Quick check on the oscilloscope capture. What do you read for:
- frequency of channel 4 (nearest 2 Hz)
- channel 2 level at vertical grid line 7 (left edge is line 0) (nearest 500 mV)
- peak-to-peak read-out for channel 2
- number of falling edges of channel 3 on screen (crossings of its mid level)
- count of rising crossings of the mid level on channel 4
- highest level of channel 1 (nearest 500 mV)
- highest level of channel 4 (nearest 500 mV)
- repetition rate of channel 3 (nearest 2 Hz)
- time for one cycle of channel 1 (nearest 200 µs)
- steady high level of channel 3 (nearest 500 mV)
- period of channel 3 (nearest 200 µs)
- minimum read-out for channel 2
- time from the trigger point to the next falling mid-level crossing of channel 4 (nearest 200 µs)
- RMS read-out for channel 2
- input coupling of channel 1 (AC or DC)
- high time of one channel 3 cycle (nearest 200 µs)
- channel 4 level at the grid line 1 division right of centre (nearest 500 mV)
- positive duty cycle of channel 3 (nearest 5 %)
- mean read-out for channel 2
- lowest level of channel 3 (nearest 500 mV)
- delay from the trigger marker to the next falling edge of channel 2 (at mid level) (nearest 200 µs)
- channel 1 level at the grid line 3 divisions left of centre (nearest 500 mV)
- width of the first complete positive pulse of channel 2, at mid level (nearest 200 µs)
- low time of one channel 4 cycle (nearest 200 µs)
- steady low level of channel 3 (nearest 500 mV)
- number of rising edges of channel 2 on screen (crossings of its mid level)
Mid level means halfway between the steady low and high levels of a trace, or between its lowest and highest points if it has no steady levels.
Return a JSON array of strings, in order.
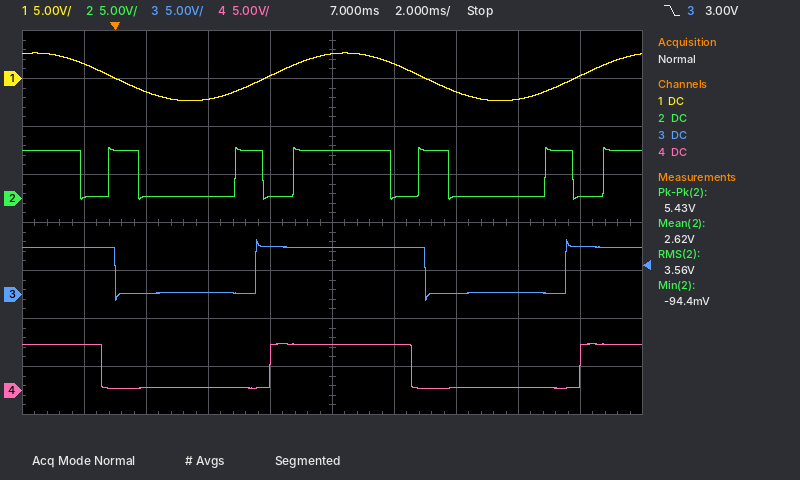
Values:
["100 Hz", "0.0 V", "5.43 V", "2", "2", "2.5 V", "5.0 V", "100 Hz", "10.0 ms", "5.0 V", "10.0 ms", "-94.4 mV", "9.6 ms", "3.56 V", "DC", "5.4 ms", "5.0 V", "55 %", "2.62 V", "-500 mV", "800 µs", "-1.5 V", "1.0 ms", "5.4 ms", "0.0 V", "6"]
